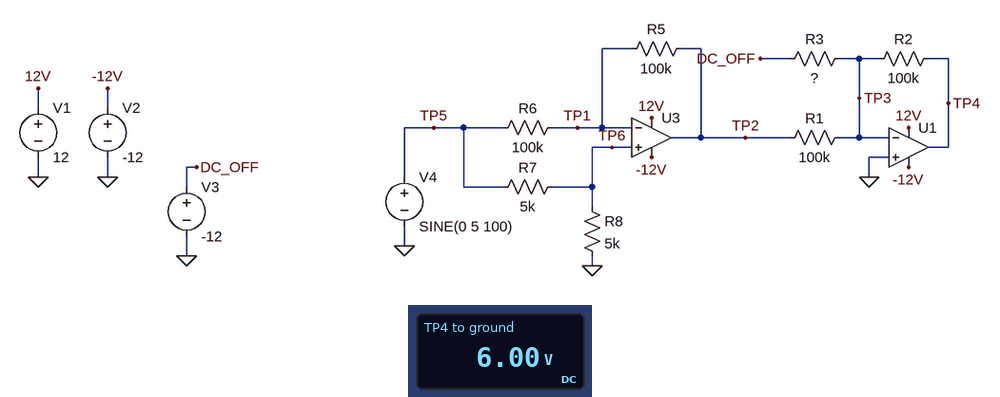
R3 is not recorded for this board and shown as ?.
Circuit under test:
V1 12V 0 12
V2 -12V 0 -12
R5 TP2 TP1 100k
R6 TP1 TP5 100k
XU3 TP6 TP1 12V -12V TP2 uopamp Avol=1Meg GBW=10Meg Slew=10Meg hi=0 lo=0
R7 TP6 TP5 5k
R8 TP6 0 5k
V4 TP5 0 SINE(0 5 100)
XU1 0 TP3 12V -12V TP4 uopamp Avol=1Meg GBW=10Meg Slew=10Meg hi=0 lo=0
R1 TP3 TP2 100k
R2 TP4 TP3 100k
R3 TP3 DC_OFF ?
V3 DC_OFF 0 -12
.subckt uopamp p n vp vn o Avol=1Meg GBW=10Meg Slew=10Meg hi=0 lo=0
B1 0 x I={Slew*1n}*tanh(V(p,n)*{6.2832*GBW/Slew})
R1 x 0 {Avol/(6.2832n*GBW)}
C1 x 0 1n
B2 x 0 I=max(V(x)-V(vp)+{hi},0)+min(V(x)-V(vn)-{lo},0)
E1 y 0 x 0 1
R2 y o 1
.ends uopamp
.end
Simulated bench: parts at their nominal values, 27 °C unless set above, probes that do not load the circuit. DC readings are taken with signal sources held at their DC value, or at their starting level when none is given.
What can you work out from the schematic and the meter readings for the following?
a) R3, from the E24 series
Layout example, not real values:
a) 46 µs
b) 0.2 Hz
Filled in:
a) 200 kΩ
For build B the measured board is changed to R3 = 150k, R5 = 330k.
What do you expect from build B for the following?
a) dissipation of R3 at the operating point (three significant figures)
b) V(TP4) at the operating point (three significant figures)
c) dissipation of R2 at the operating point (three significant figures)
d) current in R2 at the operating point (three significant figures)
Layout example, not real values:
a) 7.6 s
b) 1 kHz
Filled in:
a) 960 µW
b) 8.00 V
c) 640 µW
d) 80.0 µA
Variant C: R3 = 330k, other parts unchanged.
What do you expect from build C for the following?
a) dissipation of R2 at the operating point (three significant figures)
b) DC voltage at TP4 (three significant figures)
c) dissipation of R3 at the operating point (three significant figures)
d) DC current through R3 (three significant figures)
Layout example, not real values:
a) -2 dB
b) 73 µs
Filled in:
a) 132 µW
b) 3.64 V
c) 436 µW
d) 36.4 µA
